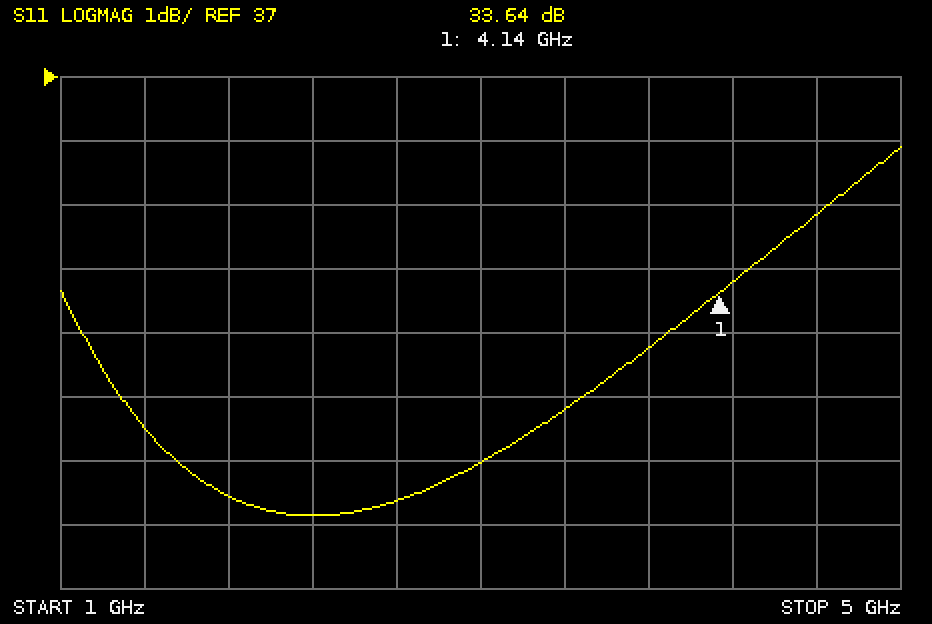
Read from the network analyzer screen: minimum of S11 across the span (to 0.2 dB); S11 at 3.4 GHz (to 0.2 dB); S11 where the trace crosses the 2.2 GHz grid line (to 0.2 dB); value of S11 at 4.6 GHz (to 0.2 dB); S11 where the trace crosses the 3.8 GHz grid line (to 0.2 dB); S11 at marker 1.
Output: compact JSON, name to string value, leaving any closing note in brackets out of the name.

{"minimum of S11 across the span": "30.2 dB", "S11 at 3.4 GHz": "31.8 dB", "S11 where the trace crosses the 2.2 GHz grid line": "30.2 dB", "value of S11 at 4.6 GHz": "34.8 dB", "S11 where the trace crosses the 3.8 GHz grid line": "32.8 dB", "S11 at marker 1": "33.64 dB"}
